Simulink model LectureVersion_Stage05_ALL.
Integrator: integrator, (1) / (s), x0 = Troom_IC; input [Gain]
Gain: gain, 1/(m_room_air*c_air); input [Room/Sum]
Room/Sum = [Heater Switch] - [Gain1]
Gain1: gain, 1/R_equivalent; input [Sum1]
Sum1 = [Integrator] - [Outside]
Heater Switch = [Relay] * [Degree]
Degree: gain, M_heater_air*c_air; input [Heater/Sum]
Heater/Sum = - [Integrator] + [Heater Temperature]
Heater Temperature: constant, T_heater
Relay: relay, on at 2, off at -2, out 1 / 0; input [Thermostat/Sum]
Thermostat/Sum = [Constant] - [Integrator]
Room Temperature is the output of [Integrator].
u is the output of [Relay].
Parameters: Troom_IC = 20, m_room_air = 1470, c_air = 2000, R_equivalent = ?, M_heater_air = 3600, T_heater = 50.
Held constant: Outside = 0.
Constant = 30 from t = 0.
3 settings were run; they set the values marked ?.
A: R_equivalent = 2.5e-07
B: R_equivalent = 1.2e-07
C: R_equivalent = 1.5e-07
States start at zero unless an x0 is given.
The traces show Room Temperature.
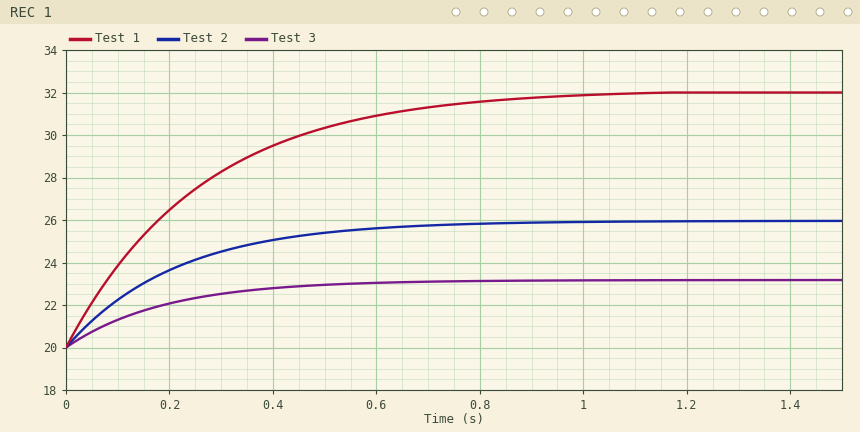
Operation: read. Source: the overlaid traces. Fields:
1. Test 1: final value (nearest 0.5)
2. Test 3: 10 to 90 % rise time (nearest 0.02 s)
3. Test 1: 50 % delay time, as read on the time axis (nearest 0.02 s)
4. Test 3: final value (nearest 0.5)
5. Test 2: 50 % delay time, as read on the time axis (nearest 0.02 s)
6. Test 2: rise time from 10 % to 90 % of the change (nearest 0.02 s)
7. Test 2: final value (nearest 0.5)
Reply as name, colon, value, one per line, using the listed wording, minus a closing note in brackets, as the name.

Test 1: final value: 32.0
Test 3: 10 to 90 % rise time: 0.42 s
Test 1: 50 % delay time, as read on the time axis: 0.18 s
Test 3: final value: 23.0
Test 2: 50 % delay time, as read on the time axis: 0.14 s
Test 2: rise time from 10 % to 90 % of the change: 0.46 s
Test 2: final value: 26.0
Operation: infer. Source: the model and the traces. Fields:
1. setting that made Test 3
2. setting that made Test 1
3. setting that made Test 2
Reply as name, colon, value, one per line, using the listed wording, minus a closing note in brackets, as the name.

setting that made Test 3: B
setting that made Test 1: A
setting that made Test 2: C
